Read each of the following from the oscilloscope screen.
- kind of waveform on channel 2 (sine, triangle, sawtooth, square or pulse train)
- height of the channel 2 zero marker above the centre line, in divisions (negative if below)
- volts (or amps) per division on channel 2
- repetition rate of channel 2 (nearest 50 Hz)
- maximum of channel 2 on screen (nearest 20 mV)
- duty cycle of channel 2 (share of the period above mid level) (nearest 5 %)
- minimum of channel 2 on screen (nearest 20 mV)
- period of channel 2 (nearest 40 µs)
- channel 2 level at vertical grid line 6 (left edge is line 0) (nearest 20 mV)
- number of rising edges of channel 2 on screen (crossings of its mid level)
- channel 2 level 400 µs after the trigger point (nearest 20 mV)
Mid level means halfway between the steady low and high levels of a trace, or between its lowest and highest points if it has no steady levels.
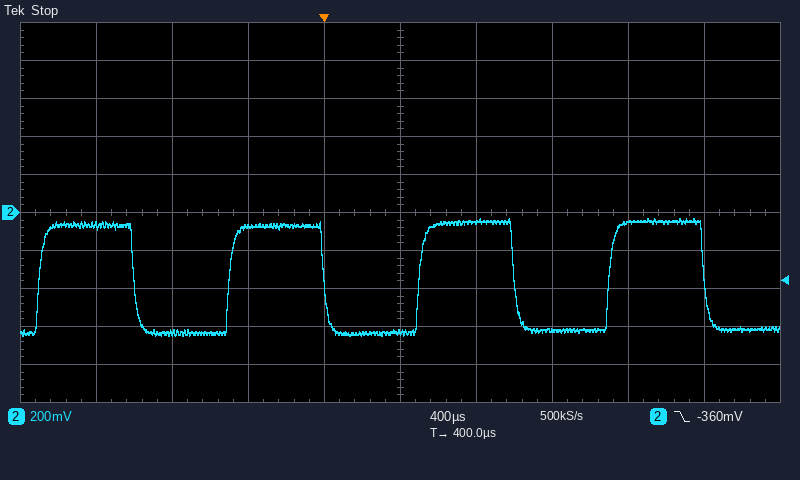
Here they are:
square
0.0 div
200 mV
1.00 kHz
-40 mV
50 %
-640 mV
1.00 ms
-40 mV
4
-640 mV
